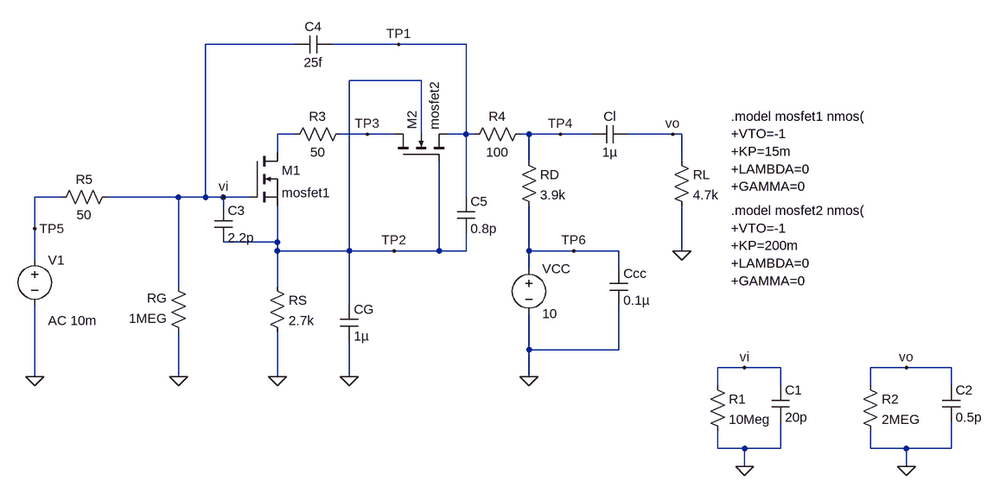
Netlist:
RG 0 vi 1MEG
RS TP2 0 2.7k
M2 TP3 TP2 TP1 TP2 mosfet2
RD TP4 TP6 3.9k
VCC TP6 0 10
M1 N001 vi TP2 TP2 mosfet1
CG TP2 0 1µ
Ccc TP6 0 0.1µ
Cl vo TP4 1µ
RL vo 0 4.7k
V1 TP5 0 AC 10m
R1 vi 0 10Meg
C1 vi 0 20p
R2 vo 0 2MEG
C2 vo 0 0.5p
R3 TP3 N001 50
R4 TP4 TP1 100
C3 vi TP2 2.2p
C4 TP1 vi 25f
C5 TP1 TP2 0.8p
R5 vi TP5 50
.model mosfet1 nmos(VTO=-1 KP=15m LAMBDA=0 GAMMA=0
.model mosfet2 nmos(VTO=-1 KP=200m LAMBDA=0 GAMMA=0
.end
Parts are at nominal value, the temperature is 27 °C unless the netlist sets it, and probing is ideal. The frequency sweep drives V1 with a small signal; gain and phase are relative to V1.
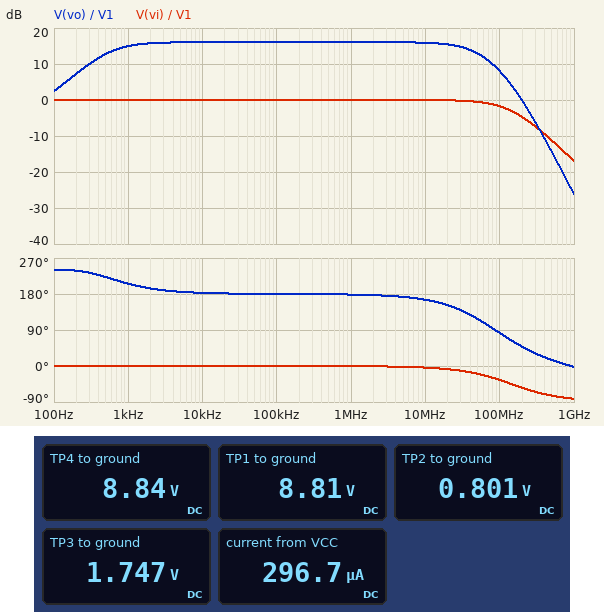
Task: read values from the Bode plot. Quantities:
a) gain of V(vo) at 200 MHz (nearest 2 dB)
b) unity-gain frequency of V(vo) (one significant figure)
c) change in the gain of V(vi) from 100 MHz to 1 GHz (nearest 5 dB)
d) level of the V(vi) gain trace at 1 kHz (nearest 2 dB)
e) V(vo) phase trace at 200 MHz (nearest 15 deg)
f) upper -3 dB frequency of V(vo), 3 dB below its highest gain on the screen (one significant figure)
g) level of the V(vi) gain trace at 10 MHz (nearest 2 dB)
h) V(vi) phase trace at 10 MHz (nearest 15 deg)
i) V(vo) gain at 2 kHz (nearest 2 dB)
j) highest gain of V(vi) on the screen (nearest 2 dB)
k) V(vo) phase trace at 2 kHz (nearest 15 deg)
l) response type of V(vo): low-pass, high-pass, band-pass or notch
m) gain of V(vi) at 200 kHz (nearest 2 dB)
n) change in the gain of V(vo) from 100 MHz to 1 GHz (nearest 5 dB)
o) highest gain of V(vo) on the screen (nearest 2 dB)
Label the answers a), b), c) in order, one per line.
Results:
a) 0 dB
b) 200 MHz
c) -15 dB
d) 0 dB
e) 45 deg
f) 50 MHz
g) 0 dB
h) 0 deg
i) 16 dB
j) 0 dB
k) 195 deg
l) band-pass
m) 0 dB
n) -35 dB
o) 16 dB
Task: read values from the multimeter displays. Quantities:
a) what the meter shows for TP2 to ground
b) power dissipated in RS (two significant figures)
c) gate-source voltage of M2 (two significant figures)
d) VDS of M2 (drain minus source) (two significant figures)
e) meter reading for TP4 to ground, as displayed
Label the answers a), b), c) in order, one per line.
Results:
a) 0.801 V
b) 240 µW
c) -8.0 V
d) -7.1 V
e) 8.84 V
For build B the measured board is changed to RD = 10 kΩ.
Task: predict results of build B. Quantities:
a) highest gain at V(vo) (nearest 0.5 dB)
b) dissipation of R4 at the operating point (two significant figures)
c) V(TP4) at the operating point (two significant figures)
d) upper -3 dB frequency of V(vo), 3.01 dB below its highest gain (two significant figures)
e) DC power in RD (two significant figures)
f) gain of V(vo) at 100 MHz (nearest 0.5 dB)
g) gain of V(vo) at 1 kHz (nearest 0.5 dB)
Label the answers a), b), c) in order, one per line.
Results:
a) 19.5 dB
b) 8.8 µW
c) 7.0 V
d) 35 MHz
e) 880 µW
f) 8.5 dB
g) 18.5 dB
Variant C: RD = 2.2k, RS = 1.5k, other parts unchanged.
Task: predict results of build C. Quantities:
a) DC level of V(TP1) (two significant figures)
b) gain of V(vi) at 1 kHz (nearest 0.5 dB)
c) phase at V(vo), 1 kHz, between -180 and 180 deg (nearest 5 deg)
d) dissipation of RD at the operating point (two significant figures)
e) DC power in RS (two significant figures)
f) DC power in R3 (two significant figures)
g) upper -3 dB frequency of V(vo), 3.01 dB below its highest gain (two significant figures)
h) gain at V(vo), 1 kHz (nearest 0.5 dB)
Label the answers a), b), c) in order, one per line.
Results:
a) 8.9 V
b) 0 dB
c) -150 deg
d) 540 µW
e) 370 µW
f) 12 µW
g) 64 MHz
h) 13.5 dB
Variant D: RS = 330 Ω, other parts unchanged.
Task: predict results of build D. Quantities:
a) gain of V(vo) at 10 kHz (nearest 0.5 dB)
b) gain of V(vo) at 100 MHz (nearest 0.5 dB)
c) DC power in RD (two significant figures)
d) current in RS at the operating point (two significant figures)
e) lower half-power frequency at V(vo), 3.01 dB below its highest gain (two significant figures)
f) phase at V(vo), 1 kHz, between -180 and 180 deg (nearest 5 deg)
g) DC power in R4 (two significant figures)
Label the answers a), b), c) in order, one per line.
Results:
a) 23.5 dB
b) 15.5 dB
c) 10 mW
d) 1.6 mA
e) 1.4 kHz
f) -145 deg
g) 260 µW
